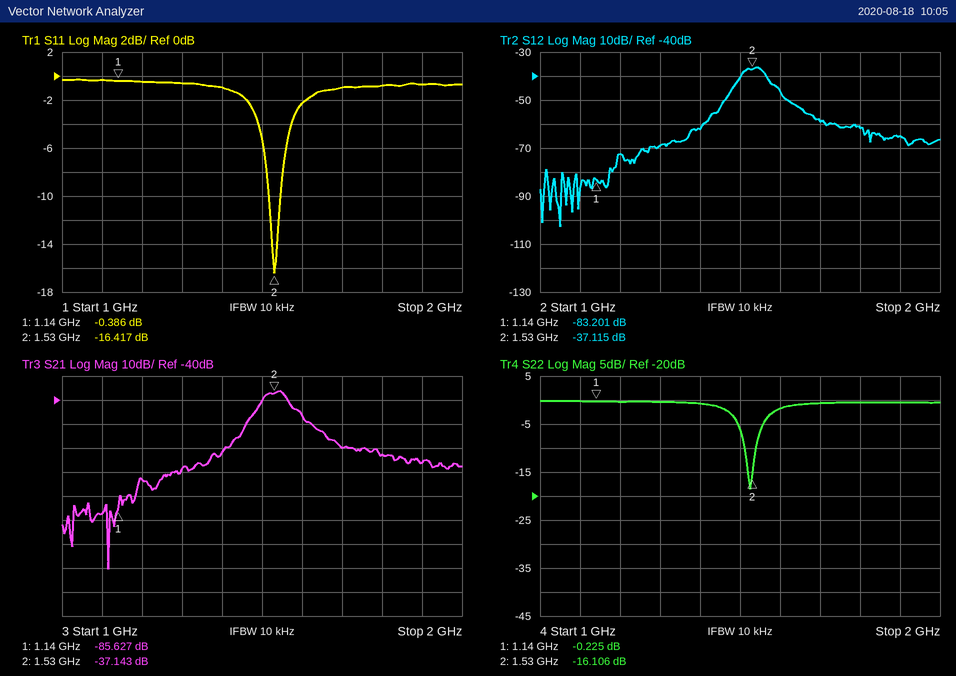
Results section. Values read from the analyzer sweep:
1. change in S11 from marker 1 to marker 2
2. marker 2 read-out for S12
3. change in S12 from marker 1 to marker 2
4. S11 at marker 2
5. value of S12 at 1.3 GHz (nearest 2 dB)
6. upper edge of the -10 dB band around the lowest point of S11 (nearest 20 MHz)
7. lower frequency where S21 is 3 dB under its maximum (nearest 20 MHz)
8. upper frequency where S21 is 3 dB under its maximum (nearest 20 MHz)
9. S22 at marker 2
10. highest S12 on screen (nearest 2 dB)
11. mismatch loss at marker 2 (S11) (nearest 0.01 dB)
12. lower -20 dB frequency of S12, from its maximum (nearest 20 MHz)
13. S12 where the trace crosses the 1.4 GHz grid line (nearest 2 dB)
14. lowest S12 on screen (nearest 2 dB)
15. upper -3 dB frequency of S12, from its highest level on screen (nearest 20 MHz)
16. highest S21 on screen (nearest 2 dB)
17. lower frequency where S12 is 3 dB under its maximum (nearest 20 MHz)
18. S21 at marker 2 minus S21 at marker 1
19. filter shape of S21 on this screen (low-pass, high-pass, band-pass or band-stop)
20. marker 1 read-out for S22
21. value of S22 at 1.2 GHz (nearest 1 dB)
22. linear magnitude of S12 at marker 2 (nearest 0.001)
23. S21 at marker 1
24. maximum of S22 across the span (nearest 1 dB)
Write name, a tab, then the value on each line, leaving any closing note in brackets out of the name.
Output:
change in S11 from marker 1 to marker 2	-16.031 dB
marker 2 read-out for S12	-37.115 dB
change in S12 from marker 1 to marker 2	46.086 dB
S11 at marker 2	-16.417 dB
value of S12 at 1.3 GHz	-68 dB
upper edge of the -10 dB band around the lowest point of S11	1.54 GHz
lower frequency where S21 is 3 dB under its maximum	1.50 GHz
upper frequency where S21 is 3 dB under its maximum	1.56 GHz
S22 at marker 2	-16.106 dB
highest S12 on screen	-36 dB
mismatch loss at marker 2 (S11)	0.10 dB
lower -20 dB frequency of S12, from its maximum	1.42 GHz
S12 where the trace crosses the 1.4 GHz grid line	-62 dB
lowest S12 on screen	-102 dB
upper -3 dB frequency of S12, from its highest level on screen	1.56 GHz
highest S21 on screen	-36 dB
lower frequency where S12 is 3 dB under its maximum	1.50 GHz
S21 at marker 2 minus S21 at marker 1	48.484 dB
filter shape of S21 on this screen	band-pass
marker 1 read-out for S22	-0.225 dB
value of S22 at 1.2 GHz	0 dB
linear magnitude of S12 at marker 2	0.014
S21 at marker 1	-85.627 dB
maximum of S22 across the span	0 dB
